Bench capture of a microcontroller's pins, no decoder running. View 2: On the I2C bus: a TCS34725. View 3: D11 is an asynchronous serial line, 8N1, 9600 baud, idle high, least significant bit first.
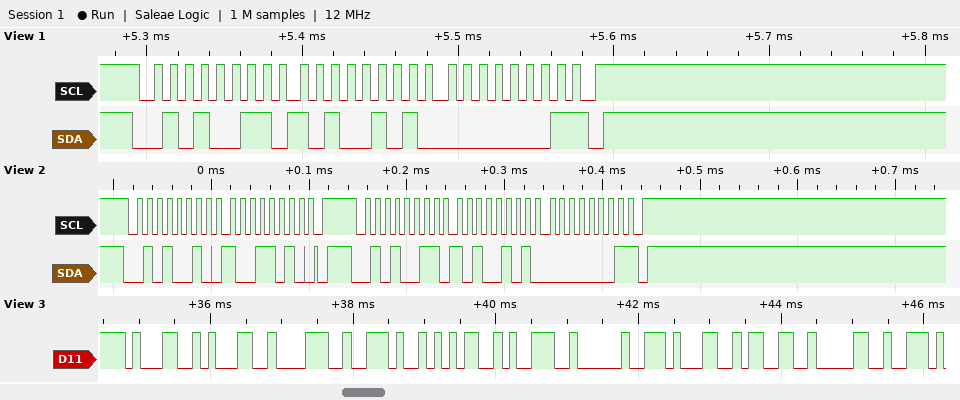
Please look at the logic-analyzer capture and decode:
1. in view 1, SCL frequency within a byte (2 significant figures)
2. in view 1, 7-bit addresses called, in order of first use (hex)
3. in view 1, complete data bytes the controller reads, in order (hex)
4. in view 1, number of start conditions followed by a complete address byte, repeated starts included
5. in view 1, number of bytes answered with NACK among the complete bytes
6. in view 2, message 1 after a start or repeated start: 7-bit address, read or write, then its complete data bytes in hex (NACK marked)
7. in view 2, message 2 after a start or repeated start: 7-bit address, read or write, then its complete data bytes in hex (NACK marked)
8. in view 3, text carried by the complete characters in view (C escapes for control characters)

100 kHz
0x29
A5 01
1
1
0x29 write: 9A
0x29 read: A5 01 NACK
"118.59 130"
